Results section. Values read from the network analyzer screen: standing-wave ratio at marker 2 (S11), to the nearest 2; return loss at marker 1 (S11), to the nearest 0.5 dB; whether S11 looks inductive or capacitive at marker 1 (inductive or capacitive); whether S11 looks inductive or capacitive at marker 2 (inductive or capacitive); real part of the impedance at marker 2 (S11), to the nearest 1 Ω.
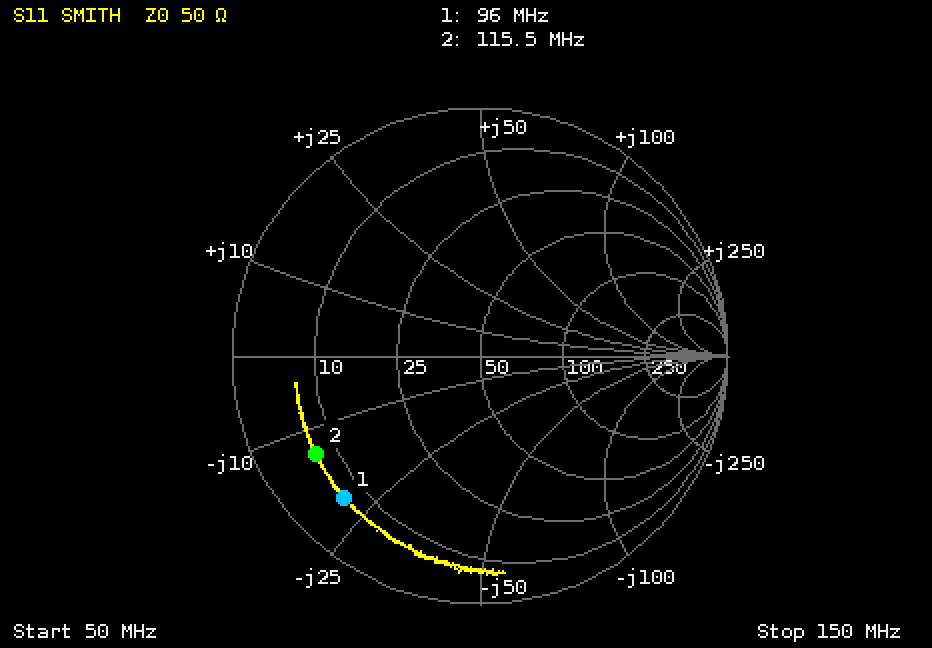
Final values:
8
2.0 dB
capacitive
capacitive
7 Ω
